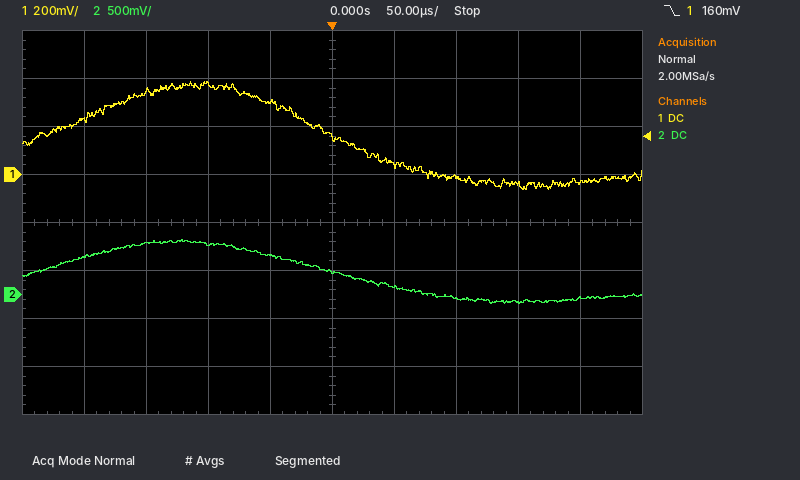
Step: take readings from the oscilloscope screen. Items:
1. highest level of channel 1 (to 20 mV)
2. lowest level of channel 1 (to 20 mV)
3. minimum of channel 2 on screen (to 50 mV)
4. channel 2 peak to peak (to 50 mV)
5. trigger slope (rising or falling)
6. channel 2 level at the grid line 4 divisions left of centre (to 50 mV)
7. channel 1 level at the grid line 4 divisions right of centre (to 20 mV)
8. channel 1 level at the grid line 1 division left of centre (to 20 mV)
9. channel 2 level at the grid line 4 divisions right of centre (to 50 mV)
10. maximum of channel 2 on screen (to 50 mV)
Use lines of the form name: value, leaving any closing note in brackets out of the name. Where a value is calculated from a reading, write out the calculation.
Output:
highest level of channel 1: 380 mV
lowest level of channel 1: -60 mV
minimum of channel 2 on screen: -100 mV
channel 2 peak to peak: 550 mV − (-100 mV) = 650 mV
trigger slope: falling
channel 2 level at the grid line 4 divisions left of centre: 400 mV
channel 1 level at the grid line 4 divisions right of centre: -40 mV
channel 1 level at the grid line 1 division left of centre: 300 mV
channel 2 level at the grid line 4 divisions right of centre: -50 mV
maximum of channel 2 on screen: 550 mV
